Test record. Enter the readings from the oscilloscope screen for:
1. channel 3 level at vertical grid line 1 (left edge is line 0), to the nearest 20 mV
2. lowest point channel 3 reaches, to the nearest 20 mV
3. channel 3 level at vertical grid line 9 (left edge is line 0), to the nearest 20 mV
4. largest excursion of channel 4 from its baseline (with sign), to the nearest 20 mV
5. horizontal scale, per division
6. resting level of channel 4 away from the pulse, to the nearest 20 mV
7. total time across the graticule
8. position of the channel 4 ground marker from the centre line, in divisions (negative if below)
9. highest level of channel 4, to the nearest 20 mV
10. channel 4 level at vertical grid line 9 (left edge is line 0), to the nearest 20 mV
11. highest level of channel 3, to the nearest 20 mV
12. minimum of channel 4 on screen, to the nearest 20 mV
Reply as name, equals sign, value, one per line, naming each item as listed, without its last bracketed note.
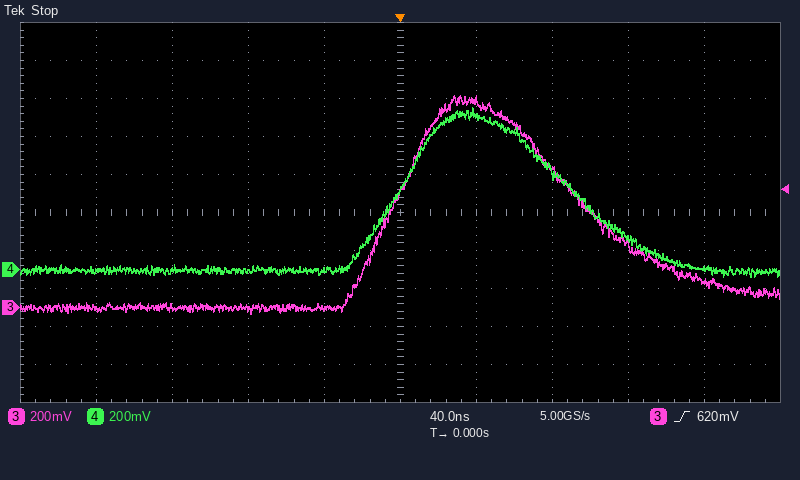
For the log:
channel 3 level at vertical grid line 1 (left edge is line 0), to the nearest 20 mV = 0 mV
lowest point channel 3 reaches, to the nearest 20 mV = -40 mV
channel 3 level at vertical grid line 9 (left edge is line 0), to the nearest 20 mV = 140 mV
largest excursion of channel 4 from its baseline (with sign), to the nearest 20 mV = +860 mV
horizontal scale, per division = 40 ns
resting level of channel 4 away from the pulse, to the nearest 20 mV = 0 mV
total time across the graticule = 400 ns
position of the channel 4 ground marker from the centre line, in divisions = -1.5 div
highest level of channel 4, to the nearest 20 mV = 860 mV
channel 4 level at vertical grid line 9 (left edge is line 0), to the nearest 20 mV = 0 mV
highest level of channel 3, to the nearest 20 mV = 1.12 V
minimum of channel 4 on screen, to the nearest 20 mV = -40 mV
